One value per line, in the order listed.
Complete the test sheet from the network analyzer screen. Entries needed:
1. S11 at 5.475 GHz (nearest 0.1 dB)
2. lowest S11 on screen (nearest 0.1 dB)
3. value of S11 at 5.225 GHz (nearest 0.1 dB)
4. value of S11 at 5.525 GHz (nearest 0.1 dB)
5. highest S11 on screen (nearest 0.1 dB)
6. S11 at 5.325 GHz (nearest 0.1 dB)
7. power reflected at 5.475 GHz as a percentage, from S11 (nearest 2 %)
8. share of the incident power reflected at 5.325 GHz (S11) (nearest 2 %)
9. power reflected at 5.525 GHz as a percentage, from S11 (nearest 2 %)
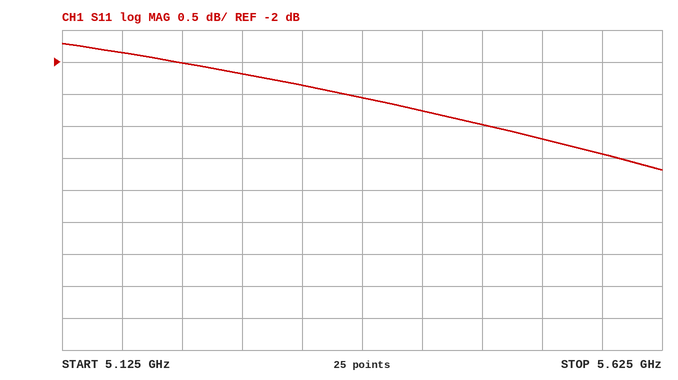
-3.0 dB
-3.7 dB
-2.0 dB
-3.2 dB
-1.7 dB
-2.4 dB
50 %
58 %
48 %
